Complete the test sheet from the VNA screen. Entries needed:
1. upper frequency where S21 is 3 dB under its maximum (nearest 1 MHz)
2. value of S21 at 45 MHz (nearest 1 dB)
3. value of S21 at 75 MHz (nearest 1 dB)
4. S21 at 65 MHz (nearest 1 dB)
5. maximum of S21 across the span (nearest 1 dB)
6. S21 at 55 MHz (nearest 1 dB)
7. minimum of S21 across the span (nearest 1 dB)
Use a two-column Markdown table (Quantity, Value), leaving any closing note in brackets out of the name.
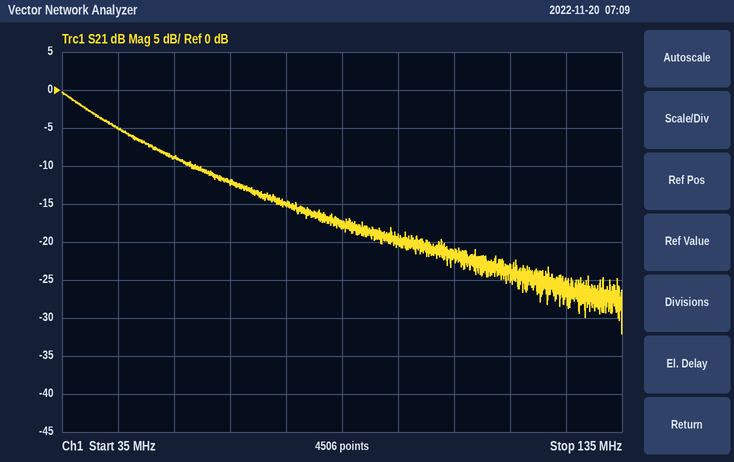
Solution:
| Quantity | Value |
|---|---|
| upper frequency where S21 is 3 dB under its maximum | 41 MHz |
| value of S21 at 45 MHz | -5 dB |
| value of S21 at 75 MHz | -15 dB |
| S21 at 65 MHz | -12 dB |
| maximum of S21 across the span | 0 dB |
| S21 at 55 MHz | -9 dB |
| minimum of S21 across the span | -32 dB |
